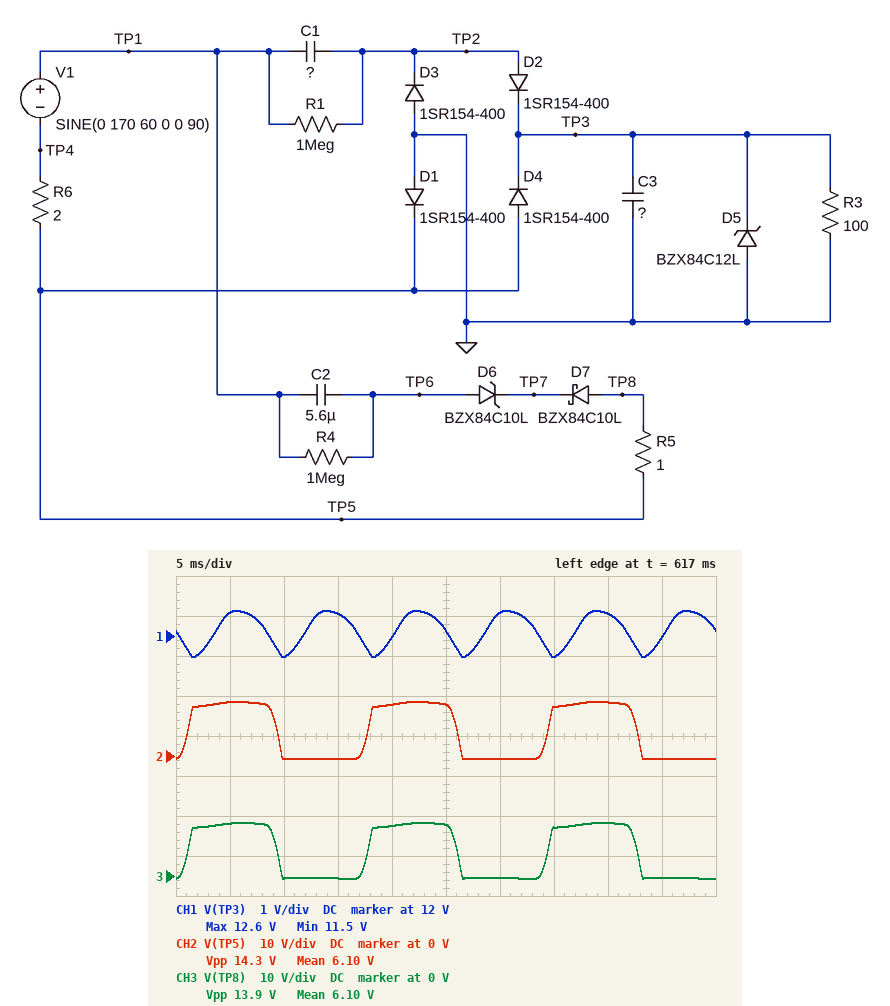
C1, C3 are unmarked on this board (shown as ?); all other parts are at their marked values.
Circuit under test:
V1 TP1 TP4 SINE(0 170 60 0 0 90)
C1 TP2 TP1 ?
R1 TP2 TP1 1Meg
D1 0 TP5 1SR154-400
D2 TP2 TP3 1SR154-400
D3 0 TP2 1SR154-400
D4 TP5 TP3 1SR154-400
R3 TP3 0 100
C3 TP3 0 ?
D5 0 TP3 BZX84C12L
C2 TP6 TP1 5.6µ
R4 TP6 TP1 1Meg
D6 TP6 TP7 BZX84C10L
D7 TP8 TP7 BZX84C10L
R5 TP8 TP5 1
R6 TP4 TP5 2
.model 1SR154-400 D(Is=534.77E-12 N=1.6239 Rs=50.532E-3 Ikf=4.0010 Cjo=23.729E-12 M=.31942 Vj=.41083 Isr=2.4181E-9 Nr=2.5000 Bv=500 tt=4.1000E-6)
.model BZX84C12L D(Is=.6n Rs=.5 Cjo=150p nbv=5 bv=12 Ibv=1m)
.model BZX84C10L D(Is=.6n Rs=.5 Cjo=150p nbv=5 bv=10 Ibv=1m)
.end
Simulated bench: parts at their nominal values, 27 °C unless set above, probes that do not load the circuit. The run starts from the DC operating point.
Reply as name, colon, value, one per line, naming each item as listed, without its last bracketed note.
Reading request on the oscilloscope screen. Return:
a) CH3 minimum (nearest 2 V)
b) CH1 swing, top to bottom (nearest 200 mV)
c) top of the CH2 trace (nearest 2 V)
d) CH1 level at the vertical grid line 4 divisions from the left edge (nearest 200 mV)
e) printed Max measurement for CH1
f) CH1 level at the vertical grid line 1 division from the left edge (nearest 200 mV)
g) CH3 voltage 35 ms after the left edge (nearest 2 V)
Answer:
CH3 minimum: 0 V
CH1 swing, top to bottom: 1.2 V
top of the CH2 trace: 14 V
CH1 level at the vertical grid line 4 divisions from the left edge: 12.0 V
printed Max measurement for CH1: 12.6 V
CH1 level at the vertical grid line 1 division from the left edge: 12.6 V
CH3 voltage 35 ms after the left edge: 12 V
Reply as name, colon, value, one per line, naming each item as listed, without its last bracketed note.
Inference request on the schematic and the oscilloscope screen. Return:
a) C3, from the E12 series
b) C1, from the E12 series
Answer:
C3, from the E12 series: 270 µF
C1, from the E12 series: 3.9 µF
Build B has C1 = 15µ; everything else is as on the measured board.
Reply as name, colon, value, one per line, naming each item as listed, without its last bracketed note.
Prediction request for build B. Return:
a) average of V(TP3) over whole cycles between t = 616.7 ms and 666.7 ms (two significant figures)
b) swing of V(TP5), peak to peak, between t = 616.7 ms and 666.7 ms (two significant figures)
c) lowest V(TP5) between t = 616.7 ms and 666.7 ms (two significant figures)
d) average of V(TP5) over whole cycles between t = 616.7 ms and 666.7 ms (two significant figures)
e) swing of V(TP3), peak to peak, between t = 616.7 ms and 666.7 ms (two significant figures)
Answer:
average of V(TP3) over whole cycles between t = 616.7 ms and 666.7 ms: 13 V
swing of V(TP5), peak to peak, between t = 616.7 ms and 666.7 ms: 15 V
lowest V(TP5) between t = 616.7 ms and 666.7 ms: -960 mV
average of V(TP5) over whole cycles between t = 616.7 ms and 666.7 ms: 6.4 V
swing of V(TP3), peak to peak, between t = 616.7 ms and 666.7 ms: 1.5 V
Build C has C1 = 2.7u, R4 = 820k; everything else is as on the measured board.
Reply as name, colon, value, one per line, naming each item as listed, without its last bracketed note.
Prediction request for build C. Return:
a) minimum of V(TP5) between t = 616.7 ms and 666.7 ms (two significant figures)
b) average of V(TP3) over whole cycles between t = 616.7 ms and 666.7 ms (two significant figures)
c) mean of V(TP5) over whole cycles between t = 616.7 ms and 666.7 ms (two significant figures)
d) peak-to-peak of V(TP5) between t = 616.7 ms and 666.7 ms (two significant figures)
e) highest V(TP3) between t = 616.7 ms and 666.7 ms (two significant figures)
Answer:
minimum of V(TP5) between t = 616.7 ms and 666.7 ms: -840 mV
average of V(TP3) over whole cycles between t = 616.7 ms and 666.7 ms: 10 V
mean of V(TP5) over whole cycles between t = 616.7 ms and 666.7 ms: 5.1 V
peak-to-peak of V(TP5) between t = 616.7 ms and 666.7 ms: 12 V
highest V(TP3) between t = 616.7 ms and 666.7 ms: 11 V
